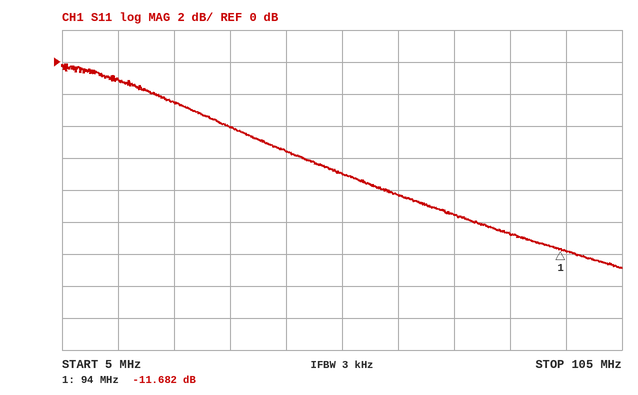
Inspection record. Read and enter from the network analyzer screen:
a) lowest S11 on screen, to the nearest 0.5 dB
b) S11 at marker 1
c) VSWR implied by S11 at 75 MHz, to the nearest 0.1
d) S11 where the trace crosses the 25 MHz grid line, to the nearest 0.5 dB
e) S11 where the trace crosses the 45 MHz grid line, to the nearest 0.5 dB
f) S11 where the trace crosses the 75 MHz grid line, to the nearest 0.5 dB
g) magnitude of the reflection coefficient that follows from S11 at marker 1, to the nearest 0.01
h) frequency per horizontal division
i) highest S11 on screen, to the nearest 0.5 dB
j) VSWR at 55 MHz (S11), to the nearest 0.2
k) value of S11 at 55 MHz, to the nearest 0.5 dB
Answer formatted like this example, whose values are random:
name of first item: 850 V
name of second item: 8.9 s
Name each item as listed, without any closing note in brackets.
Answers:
lowest S11 on screen, to the nearest 0.5 dB: -13.0 dB
S11 at marker 1: -11.682 dB
VSWR implied by S11 at 75 MHz, to the nearest 0.1: 2.0
S11 where the trace crosses the 25 MHz grid line, to the nearest 0.5 dB: -2.5 dB
S11 where the trace crosses the 45 MHz grid line, to the nearest 0.5 dB: -5.5 dB
S11 where the trace crosses the 75 MHz grid line, to the nearest 0.5 dB: -9.5 dB
magnitude of the reflection coefficient that follows from S11 at marker 1, to the nearest 0.01: 0.26
frequency per horizontal division: 10 MHz
highest S11 on screen, to the nearest 0.5 dB: 0.0 dB
VSWR at 55 MHz (S11), to the nearest 0.2: 2.6
value of S11 at 55 MHz, to the nearest 0.5 dB: -7.0 dB
